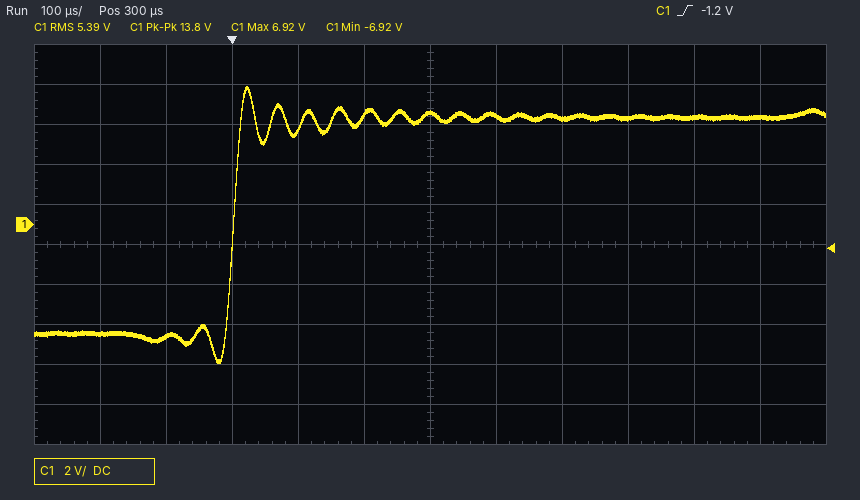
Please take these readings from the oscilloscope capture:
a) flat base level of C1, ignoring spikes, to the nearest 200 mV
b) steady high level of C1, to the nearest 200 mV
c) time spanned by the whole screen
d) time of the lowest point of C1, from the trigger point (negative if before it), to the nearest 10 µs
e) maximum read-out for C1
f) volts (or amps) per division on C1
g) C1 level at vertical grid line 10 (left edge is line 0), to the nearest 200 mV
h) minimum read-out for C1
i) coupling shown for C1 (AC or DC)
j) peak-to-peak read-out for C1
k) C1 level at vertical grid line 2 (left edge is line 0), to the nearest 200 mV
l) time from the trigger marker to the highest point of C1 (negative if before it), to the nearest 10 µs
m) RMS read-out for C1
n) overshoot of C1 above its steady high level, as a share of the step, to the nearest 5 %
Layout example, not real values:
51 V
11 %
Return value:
-5.4 V
5.4 V
1.2 ms
-20 µs
6.92 V
2 V
5.4 V
-6.92 V
DC
13.8 V
-5.6 V
+20 µs
5.39 V
15 %
